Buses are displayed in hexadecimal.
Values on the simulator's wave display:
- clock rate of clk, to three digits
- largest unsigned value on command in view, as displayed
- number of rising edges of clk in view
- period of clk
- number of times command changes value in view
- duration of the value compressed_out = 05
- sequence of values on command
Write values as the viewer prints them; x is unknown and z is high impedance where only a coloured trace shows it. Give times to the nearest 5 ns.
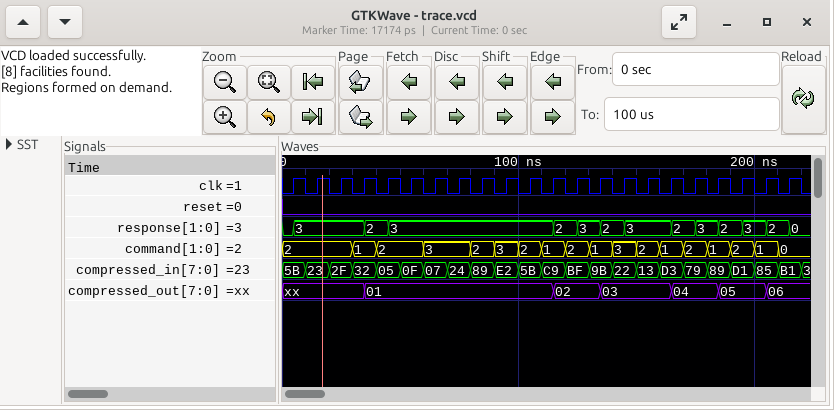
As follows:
100 MHz
3
22
10 ns
17
20 ns
2, 1, 2, 3, 2, 3, 2, 1, 2, 1, 3, 2, 1, 2, 1, 2, 1, 0
